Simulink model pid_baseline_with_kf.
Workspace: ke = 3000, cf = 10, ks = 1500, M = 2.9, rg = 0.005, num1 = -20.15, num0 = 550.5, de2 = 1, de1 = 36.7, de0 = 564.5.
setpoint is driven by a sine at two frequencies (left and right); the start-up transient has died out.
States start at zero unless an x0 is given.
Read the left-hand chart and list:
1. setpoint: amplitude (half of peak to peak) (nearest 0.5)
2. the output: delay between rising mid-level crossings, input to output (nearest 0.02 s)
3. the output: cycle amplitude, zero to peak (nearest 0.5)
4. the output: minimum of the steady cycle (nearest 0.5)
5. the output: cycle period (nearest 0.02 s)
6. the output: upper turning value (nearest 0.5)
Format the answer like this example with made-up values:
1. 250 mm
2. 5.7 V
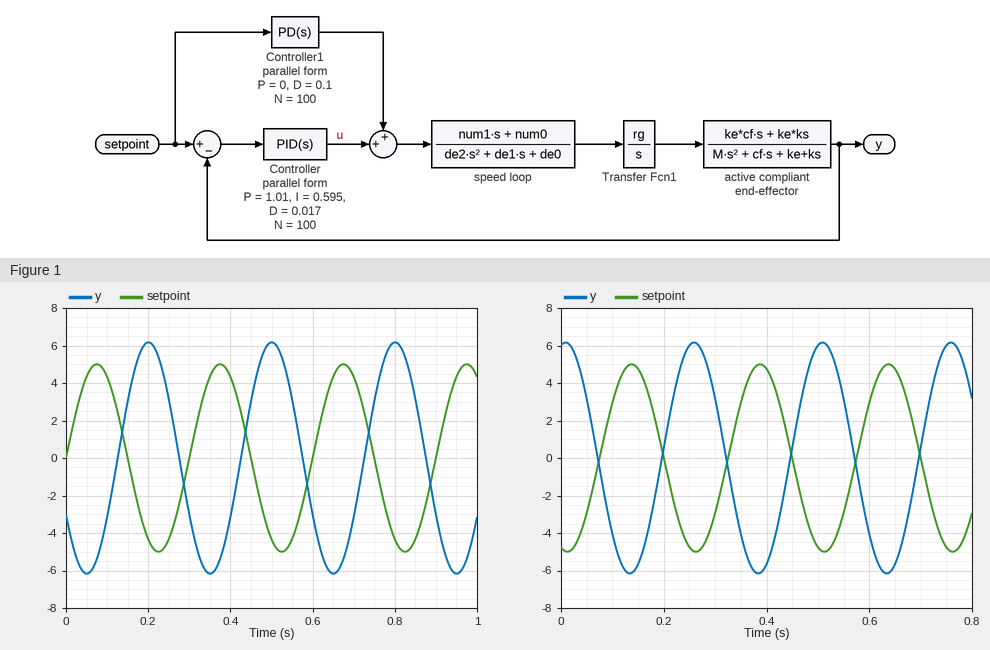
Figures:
1. 5.0
2. 0.12 s
3. 6.0
4. -6.0
5. 0.30 s
6. 6.0
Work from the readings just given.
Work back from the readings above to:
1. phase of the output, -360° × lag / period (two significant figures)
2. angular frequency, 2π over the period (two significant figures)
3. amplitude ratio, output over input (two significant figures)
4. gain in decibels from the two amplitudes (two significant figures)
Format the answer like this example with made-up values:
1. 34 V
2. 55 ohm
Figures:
1. -140°
2. 21 rad/s
3. 1.2
4. 1.6 dB
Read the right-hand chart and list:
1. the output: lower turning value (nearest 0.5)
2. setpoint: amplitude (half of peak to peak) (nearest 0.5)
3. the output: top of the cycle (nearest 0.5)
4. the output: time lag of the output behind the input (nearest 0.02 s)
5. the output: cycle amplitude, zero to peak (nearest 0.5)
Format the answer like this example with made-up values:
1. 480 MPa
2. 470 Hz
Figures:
1. -6.0
2. 5.0
3. 6.0
4. 0.12 s
5. 6.0
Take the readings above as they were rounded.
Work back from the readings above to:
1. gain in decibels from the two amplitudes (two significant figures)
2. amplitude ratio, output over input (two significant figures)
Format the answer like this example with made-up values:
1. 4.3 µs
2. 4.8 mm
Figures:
1. 1.6 dB
2. 1.2
